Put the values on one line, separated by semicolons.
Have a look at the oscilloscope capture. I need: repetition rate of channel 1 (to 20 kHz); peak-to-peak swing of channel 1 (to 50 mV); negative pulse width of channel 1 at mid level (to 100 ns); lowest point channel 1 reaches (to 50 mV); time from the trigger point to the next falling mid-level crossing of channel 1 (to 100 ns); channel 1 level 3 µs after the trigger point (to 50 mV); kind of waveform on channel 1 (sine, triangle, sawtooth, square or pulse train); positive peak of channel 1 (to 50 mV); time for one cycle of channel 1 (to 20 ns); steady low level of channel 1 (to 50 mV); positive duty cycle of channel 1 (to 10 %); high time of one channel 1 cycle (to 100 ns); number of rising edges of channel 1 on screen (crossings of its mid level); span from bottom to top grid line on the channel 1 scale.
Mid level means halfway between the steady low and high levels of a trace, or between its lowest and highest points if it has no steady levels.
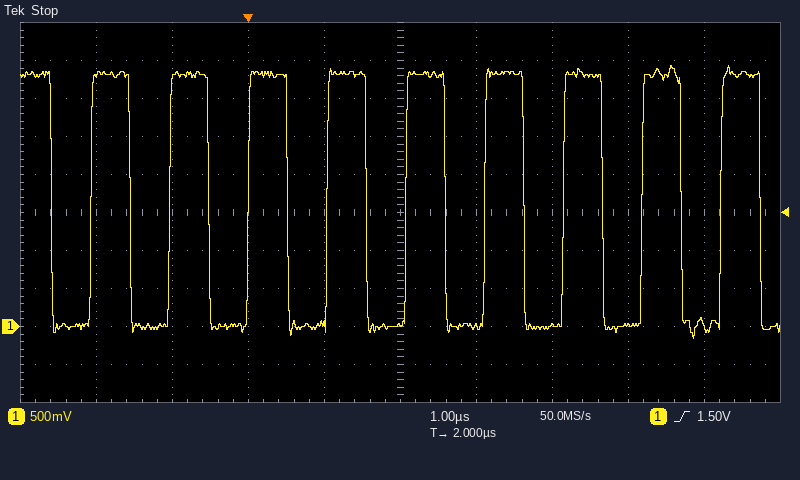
960 kHz; 3.60 V; 500 ns; -150 mV; 500 ns; 0 mV; square; 3.45 V; 1.04 µs; 0 mV; 50 %; 500 ns; 9; 5 V
